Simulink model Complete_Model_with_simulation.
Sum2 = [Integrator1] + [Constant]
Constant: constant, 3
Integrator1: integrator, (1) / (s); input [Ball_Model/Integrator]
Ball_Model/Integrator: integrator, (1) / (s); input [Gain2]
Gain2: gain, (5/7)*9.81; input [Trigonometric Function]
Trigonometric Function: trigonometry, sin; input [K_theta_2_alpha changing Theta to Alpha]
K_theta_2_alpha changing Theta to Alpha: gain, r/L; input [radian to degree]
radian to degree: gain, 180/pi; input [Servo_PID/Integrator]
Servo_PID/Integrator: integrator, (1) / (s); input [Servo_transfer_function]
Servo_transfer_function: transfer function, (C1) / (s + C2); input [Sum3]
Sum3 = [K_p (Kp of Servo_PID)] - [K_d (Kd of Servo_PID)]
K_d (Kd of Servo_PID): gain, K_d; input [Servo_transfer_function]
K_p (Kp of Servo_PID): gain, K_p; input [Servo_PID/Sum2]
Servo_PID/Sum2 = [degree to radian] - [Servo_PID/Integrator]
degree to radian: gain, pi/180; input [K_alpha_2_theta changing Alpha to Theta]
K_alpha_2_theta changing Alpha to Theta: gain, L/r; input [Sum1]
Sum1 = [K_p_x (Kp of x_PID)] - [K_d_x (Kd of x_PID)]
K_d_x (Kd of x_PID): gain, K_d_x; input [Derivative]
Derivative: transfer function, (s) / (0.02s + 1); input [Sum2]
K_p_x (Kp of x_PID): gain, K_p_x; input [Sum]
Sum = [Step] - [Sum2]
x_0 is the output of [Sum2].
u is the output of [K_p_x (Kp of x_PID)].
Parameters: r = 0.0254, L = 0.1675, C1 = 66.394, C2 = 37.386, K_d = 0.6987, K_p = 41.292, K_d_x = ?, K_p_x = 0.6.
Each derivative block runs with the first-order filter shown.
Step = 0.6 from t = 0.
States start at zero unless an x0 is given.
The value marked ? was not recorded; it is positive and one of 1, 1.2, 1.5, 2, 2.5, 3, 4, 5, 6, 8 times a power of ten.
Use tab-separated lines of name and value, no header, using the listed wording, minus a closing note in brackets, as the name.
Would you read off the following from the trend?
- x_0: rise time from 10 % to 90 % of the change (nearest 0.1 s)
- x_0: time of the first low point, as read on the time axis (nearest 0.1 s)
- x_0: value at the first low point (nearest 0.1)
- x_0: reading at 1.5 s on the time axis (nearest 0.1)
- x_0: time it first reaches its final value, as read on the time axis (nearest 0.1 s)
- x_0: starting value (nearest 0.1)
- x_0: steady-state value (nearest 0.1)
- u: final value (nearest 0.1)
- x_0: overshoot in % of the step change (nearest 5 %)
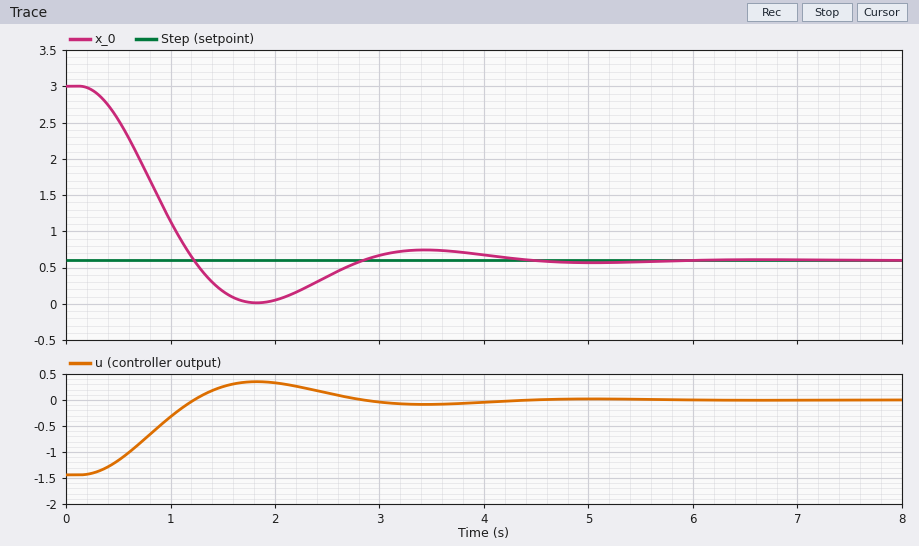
x_0: rise time from 10 % to 90 % of the change	0.7 s
x_0: time of the first low point, as read on the time axis	1.8 s
x_0: value at the first low point	0.0
x_0: reading at 1.5 s on the time axis	0.2
x_0: time it first reaches its final value, as read on the time axis	1.2 s
x_0: starting value	3.0
x_0: steady-state value	0.6
u: final value	0.0
x_0: overshoot in % of the step change	25 %
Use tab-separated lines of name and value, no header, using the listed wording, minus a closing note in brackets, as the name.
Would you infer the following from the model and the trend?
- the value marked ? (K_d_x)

the value marked ?	0.25
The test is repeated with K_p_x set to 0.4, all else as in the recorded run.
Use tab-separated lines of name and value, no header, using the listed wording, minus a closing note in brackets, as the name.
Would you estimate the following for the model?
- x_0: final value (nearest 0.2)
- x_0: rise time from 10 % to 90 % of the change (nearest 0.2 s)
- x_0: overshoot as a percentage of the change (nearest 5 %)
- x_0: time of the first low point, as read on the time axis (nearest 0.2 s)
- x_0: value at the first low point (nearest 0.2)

x_0: final value	0.6
x_0: rise time from 10 % to 90 % of the change	1.0 s
x_0: overshoot as a percentage of the change	15 %
x_0: time of the first low point, as read on the time axis	2.2 s
x_0: value at the first low point	0.2
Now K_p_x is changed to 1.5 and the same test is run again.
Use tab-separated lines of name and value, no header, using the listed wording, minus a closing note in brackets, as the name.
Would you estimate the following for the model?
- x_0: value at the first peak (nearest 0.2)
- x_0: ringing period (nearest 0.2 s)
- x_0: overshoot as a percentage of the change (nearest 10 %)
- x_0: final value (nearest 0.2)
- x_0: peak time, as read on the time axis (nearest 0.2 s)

x_0: value at the first peak	5.6
x_0: ringing period	2.0 s
x_0: overshoot as a percentage of the change	50 %
x_0: final value	4.8
x_0: peak time, as read on the time axis	1.6 s
